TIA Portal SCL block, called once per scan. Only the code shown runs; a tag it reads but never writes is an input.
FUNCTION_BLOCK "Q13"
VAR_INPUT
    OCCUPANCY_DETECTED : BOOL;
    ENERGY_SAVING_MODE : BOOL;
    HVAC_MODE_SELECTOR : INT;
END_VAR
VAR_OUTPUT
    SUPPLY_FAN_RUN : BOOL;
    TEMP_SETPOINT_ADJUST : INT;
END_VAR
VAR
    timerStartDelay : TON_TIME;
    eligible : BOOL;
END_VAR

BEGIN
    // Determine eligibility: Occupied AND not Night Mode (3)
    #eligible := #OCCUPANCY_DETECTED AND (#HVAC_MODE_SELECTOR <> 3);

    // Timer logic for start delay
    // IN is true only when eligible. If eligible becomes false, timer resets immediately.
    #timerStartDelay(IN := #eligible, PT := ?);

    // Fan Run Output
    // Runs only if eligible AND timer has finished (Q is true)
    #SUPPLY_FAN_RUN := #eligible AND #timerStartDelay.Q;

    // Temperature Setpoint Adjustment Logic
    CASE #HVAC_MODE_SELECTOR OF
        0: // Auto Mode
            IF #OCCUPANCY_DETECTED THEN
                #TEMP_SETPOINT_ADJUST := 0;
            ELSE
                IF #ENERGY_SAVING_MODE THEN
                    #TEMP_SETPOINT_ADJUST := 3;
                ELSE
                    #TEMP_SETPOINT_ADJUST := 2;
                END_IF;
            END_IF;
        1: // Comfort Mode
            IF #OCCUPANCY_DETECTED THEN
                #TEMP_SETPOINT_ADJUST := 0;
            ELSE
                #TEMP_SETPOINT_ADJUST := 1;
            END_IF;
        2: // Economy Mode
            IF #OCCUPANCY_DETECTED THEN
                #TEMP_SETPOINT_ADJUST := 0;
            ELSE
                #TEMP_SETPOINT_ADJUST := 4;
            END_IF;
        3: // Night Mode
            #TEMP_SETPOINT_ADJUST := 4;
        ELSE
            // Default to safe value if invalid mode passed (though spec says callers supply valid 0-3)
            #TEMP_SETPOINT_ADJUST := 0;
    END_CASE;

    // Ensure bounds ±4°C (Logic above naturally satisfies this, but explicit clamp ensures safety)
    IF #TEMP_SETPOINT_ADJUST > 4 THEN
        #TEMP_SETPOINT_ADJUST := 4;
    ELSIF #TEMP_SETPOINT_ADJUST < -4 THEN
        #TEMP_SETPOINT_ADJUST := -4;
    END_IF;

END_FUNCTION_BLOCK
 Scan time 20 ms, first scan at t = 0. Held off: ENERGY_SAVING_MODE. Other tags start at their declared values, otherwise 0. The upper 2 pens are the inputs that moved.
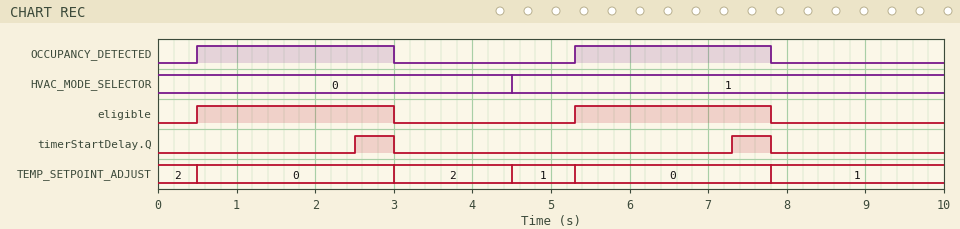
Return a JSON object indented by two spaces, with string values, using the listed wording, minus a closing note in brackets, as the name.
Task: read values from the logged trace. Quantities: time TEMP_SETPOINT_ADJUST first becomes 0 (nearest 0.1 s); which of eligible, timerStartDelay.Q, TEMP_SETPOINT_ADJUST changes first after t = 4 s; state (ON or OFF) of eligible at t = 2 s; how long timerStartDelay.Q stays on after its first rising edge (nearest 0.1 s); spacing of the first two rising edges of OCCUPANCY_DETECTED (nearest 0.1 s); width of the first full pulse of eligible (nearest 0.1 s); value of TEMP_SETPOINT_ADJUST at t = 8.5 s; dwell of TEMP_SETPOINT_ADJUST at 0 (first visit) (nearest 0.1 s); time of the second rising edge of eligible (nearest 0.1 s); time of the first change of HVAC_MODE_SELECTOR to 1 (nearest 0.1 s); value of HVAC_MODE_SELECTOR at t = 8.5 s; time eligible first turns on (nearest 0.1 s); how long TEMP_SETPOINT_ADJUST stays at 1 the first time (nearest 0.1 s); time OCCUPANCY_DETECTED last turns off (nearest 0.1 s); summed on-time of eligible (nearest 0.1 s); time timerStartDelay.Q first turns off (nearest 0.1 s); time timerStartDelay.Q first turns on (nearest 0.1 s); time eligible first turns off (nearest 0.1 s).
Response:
{
  "time TEMP_SETPOINT_ADJUST first becomes 0": "0.5 s",
  "which of eligible, timerStartDelay.Q, TEMP_SETPOINT_ADJUST changes first after t = 4 s": "TEMP_SETPOINT_ADJUST",
  "state (ON or OFF) of eligible at t = 2 s": "ON",
  "how long timerStartDelay.Q stays on after its first rising edge": "0.5 s",
  "spacing of the first two rising edges of OCCUPANCY_DETECTED": "4.8 s",
  "width of the first full pulse of eligible": "2.5 s",
  "value of TEMP_SETPOINT_ADJUST at t = 8.5 s": "1",
  "dwell of TEMP_SETPOINT_ADJUST at 0 (first visit)": "2.5 s",
  "time of the second rising edge of eligible": "5.3 s",
  "time of the first change of HVAC_MODE_SELECTOR to 1": "4.5 s",
  "value of HVAC_MODE_SELECTOR at t = 8.5 s": "1",
  "time eligible first turns on": "0.5 s",
  "how long TEMP_SETPOINT_ADJUST stays at 1 the first time": "0.8 s",
  "time OCCUPANCY_DETECTED last turns off": "7.8 s",
  "summed on-time of eligible": "5.0 s",
  "time timerStartDelay.Q first turns off": "3.0 s",
  "time timerStartDelay.Q first turns on": "2.5 s",
  "time eligible first turns off": "3.0 s"
}
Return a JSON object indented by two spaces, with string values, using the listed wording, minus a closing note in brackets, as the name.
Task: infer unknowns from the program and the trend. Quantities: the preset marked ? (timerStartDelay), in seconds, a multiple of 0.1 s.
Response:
{
  "the preset marked ? (timerStartDelay), in seconds, a multiple of 0.1 s": "2.0 s"
}
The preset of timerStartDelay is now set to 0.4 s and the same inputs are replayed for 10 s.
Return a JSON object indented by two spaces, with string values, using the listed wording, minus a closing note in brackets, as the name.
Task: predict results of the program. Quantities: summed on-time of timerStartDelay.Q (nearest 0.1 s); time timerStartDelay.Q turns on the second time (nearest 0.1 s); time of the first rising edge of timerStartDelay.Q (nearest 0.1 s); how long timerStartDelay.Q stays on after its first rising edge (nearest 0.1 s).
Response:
{
  "summed on-time of timerStartDelay.Q": "4.2 s",
  "time timerStartDelay.Q turns on the second time": "5.7 s",
  "time of the first rising edge of timerStartDelay.Q": "0.9 s",
  "how long timerStartDelay.Q stays on after its first rising edge": "2.1 s"
}
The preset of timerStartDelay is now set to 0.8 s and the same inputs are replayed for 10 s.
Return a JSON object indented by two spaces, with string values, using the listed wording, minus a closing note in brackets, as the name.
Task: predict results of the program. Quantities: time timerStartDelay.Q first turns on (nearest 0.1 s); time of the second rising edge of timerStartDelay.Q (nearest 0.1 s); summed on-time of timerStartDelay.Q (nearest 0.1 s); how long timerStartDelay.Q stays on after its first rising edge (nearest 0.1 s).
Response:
{
  "time timerStartDelay.Q first turns on": "1.3 s",
  "time of the second rising edge of timerStartDelay.Q": "6.1 s",
  "summed on-time of timerStartDelay.Q": "3.4 s",
  "how long timerStartDelay.Q stays on after its first rising edge": "1.7 s"
}
